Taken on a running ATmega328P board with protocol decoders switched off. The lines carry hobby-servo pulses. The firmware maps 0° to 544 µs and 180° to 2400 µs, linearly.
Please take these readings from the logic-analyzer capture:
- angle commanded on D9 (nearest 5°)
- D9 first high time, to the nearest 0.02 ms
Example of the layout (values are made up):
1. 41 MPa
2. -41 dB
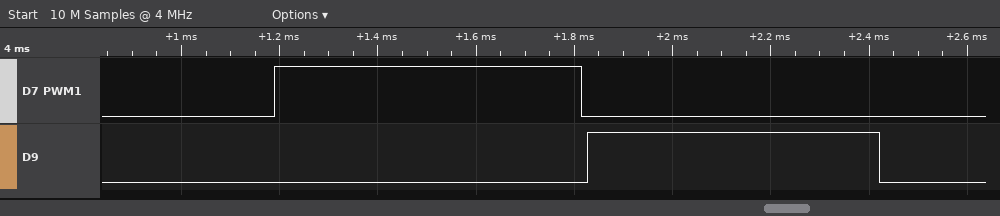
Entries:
1. 5°
2. 0.60 ms
